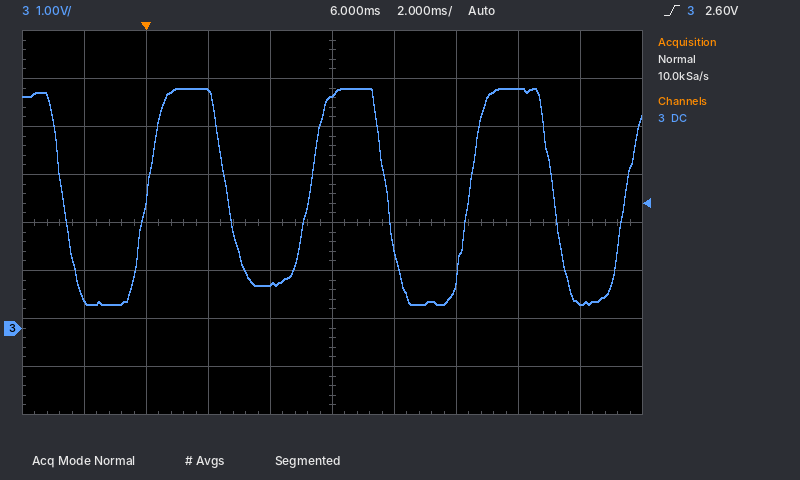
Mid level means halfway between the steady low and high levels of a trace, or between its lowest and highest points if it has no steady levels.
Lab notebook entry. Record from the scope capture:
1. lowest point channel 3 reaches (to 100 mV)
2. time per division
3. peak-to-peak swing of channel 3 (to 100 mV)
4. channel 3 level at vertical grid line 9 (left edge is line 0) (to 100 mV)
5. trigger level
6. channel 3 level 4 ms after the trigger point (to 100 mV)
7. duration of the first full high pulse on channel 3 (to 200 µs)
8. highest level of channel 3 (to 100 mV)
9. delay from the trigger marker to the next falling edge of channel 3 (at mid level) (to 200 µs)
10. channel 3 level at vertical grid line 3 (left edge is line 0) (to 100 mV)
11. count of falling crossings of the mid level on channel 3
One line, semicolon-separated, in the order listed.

500 mV; 2 ms; 4.5 V; 500 mV; 2.60 V; 900 mV; 2.6 ms; 5.0 V; 2.6 ms; 4.9 V; 4
